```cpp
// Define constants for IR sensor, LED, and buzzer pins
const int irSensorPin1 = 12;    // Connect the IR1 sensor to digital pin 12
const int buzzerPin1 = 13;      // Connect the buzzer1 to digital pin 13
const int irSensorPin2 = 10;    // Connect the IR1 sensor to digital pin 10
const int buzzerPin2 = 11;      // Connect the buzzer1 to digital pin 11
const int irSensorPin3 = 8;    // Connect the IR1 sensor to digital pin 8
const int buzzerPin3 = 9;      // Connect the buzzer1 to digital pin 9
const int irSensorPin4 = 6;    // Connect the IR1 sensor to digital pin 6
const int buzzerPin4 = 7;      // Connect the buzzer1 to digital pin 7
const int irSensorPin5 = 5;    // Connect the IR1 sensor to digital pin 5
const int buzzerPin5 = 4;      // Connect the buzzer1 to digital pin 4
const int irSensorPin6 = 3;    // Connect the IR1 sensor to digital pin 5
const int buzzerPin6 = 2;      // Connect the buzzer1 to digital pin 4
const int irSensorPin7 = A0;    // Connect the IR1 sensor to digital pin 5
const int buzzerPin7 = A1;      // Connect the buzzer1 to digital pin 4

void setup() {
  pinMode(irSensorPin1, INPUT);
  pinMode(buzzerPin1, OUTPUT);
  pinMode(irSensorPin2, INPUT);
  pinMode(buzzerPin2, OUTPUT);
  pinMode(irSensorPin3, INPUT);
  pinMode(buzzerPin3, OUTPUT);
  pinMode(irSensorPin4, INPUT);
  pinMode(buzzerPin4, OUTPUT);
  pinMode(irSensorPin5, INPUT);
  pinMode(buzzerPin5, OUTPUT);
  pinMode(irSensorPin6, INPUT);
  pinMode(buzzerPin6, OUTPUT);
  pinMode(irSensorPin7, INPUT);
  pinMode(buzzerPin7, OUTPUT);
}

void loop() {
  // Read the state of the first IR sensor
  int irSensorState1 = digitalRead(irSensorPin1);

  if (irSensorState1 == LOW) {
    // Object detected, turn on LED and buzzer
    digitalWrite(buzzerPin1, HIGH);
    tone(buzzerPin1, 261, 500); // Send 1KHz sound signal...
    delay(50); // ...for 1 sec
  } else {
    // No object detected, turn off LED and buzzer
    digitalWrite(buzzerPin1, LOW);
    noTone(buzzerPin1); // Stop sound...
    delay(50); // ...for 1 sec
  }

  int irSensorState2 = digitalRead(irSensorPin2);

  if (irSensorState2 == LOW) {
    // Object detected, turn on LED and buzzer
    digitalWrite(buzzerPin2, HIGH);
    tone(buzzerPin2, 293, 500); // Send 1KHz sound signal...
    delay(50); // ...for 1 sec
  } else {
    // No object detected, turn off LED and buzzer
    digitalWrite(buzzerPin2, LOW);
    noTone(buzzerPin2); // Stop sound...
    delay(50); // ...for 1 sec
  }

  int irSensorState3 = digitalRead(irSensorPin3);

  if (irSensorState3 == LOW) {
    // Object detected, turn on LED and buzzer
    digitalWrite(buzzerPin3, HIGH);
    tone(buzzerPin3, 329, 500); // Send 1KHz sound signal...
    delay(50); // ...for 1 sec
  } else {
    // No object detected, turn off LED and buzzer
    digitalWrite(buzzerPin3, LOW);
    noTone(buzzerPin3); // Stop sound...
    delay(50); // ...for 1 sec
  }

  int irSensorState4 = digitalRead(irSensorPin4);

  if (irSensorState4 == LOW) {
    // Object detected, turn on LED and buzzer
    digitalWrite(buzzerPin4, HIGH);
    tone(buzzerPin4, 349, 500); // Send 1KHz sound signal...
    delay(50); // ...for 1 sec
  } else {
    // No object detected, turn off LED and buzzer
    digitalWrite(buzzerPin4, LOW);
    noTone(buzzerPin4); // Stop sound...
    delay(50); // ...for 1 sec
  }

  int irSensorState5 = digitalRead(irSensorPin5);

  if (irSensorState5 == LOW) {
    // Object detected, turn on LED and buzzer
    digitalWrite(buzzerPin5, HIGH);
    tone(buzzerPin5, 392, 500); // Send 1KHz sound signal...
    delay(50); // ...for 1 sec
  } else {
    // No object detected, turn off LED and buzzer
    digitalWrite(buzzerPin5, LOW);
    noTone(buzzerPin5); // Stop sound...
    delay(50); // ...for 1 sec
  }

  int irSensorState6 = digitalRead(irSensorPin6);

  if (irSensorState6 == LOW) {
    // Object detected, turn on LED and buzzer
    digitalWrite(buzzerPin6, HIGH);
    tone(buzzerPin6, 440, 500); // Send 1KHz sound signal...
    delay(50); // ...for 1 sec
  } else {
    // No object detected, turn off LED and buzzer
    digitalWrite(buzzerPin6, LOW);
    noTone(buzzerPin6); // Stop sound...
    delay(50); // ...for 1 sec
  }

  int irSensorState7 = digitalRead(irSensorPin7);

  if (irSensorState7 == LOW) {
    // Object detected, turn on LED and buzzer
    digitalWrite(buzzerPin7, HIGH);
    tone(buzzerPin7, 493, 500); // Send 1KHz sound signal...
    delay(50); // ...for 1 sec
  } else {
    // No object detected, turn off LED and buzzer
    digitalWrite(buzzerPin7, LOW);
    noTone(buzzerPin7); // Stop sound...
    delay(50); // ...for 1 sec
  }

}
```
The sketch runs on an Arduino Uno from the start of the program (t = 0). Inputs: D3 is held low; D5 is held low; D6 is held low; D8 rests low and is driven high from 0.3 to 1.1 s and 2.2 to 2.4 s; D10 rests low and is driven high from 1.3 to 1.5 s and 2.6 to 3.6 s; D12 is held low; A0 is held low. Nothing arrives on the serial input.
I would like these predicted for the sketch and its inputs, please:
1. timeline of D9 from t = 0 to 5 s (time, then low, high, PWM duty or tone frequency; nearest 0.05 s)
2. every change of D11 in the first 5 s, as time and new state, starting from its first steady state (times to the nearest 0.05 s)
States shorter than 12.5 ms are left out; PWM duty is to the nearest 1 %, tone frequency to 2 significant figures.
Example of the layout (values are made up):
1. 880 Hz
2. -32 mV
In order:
1. 0 s low; 0.1 s high; 0.45 s low; 1.15 s high; 2.2 s low; 2.55 s high
2. 0 s low; 0.05 s high; 1.45 s low; 1.8 s high; 2.85 s low; 3.9 s high
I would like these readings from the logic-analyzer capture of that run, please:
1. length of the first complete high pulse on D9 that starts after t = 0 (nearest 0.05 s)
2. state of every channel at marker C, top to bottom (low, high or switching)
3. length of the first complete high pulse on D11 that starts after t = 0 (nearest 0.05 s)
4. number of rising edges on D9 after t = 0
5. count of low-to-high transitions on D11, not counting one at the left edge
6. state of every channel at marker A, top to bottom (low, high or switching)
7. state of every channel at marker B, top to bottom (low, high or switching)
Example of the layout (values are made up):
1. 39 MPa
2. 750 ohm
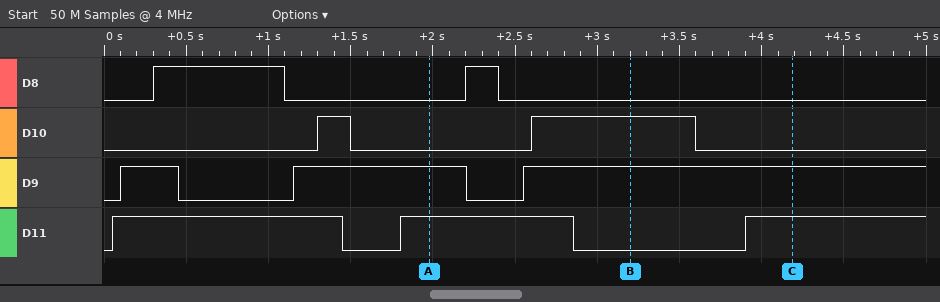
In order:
1. 0.35 s
2. D8 low, D10 low, D9 high, D11 high
3. 1.40 s
4. 3
5. 3
6. D8 low, D10 low, D9 high, D11 high
7. D8 low, D10 high, D9 high, D11 low
